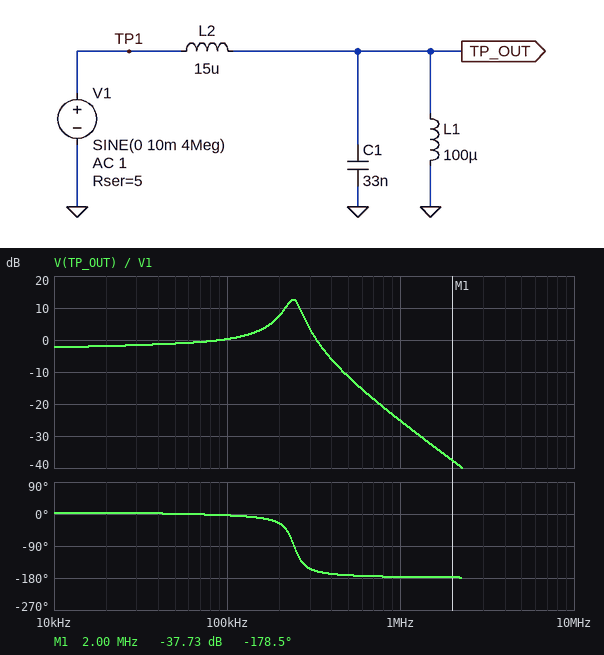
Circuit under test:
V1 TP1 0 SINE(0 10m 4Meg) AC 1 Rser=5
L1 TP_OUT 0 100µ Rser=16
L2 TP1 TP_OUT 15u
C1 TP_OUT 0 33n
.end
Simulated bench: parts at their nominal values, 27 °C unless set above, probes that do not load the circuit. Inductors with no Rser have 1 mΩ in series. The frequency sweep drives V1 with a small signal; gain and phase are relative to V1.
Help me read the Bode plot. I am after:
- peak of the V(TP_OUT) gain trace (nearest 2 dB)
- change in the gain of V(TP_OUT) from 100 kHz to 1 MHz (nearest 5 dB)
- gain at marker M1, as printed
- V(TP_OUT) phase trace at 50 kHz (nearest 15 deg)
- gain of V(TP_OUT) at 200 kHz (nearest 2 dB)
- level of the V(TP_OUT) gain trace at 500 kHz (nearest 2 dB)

12 dB
-25 dB
-37.73 dB
0 deg
8 dB
-12 dB
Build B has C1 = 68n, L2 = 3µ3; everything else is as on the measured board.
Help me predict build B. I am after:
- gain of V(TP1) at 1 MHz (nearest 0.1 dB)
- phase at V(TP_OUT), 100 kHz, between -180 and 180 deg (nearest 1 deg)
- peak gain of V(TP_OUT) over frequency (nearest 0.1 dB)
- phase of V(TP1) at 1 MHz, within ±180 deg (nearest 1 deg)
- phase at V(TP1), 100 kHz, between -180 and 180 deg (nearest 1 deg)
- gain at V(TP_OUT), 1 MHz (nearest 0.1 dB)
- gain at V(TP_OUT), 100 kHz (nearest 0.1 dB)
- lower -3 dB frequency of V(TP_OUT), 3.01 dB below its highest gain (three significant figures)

-0.3 dB
-9 deg
3.6 dB
15 deg
-8 deg
-18.2 dB
0.2 dB
122 kHz
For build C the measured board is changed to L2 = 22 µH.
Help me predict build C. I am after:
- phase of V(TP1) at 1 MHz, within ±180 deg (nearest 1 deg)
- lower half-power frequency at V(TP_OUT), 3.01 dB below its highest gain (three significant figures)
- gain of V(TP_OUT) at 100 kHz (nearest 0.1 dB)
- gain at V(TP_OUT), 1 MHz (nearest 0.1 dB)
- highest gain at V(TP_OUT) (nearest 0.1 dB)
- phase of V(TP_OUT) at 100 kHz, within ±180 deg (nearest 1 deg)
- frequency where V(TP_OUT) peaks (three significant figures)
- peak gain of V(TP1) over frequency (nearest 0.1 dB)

2 deg
187 kHz
0.5 dB
-28.8 dB
13.9 dB
-5 deg
205 kHz
0 dB
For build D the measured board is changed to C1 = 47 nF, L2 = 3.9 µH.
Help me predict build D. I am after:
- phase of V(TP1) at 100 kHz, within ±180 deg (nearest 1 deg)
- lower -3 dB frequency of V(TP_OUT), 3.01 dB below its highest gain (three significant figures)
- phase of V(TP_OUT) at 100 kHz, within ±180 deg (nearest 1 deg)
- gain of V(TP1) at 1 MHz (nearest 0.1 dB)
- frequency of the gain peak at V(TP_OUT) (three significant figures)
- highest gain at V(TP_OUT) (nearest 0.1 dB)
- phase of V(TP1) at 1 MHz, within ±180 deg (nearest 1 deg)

-4 deg
227 kHz
-5 deg
-0.2 dB
351 kHz
5.7 dB
13 deg
